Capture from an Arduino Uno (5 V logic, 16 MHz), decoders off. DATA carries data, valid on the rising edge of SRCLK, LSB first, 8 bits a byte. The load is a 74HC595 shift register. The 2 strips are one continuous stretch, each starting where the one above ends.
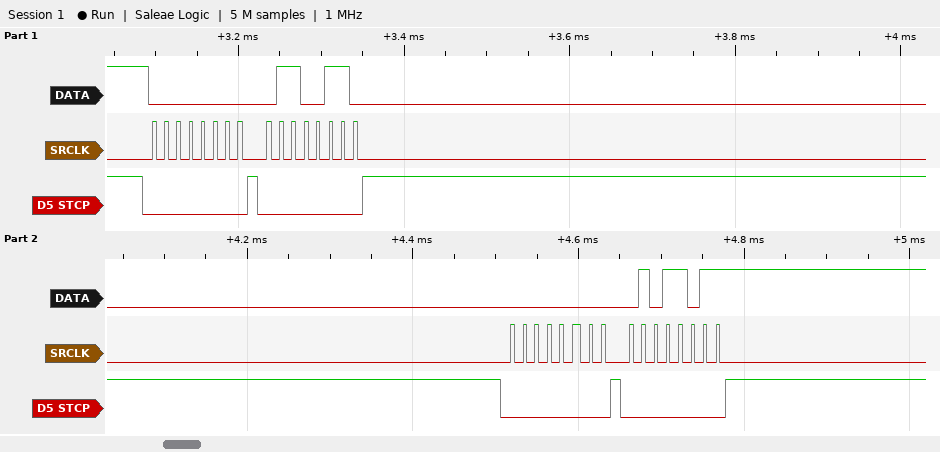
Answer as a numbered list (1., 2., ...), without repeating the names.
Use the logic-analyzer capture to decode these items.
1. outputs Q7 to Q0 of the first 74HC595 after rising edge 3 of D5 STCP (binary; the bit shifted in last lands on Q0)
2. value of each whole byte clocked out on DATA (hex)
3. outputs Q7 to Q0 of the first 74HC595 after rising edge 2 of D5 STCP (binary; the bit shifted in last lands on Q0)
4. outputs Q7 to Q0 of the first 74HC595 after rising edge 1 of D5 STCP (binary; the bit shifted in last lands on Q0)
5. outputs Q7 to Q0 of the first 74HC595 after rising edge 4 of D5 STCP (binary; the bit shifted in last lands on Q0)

1. 00000000
2. 0x00 0x66 0x00 0xDA
3. 01100110
4. 00000000
5. 01011011
